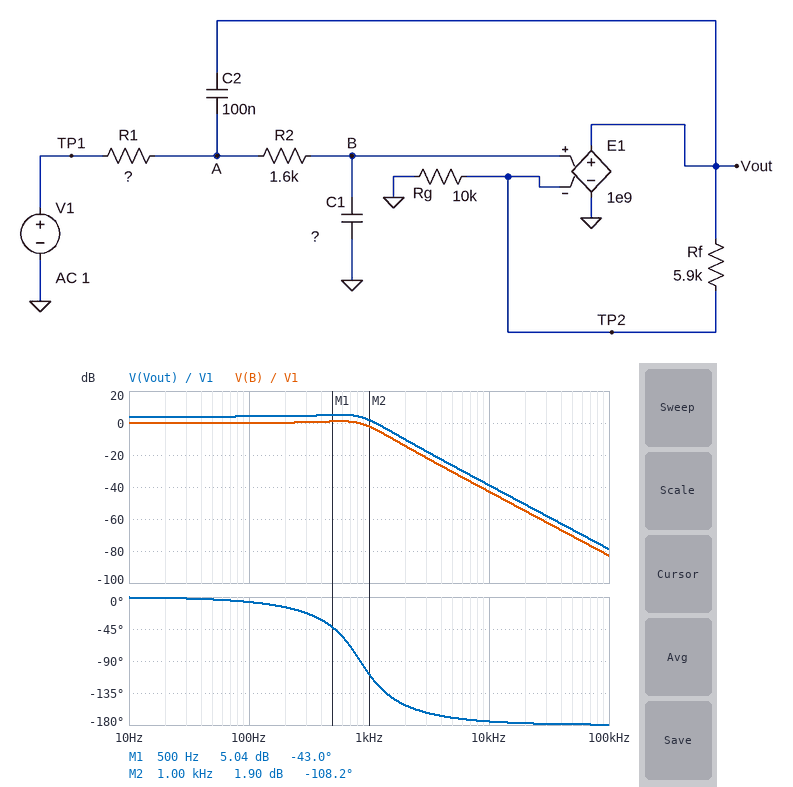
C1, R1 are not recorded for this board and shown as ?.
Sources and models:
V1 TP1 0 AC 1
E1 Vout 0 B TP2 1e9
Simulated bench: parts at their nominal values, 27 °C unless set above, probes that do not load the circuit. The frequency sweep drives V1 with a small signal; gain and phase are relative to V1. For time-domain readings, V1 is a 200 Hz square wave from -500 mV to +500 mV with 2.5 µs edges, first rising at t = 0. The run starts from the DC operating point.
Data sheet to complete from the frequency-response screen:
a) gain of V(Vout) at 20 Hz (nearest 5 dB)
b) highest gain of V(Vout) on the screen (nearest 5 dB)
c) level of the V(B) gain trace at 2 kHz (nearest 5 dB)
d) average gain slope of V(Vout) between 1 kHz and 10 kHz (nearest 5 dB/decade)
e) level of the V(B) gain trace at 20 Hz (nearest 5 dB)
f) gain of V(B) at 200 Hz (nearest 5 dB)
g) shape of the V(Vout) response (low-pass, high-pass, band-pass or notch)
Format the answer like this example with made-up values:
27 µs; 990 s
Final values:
5 dB; 5 dB; -15 dB; -40 dB/decade; 0 dB; 0 dB; low-pass
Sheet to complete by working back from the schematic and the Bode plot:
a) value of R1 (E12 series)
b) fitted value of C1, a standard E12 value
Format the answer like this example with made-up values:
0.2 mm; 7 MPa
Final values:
2.7 kΩ; 82 nF
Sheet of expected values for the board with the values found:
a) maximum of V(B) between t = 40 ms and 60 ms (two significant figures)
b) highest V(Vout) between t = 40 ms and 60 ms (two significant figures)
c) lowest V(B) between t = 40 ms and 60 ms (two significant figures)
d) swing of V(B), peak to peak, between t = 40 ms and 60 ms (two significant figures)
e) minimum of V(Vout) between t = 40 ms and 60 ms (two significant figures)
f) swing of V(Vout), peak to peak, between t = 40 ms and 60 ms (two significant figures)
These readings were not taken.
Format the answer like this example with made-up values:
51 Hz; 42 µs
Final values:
650 mV; 1.0 V; -650 mV; 1.3 V; -1.0 V; 2.1 V
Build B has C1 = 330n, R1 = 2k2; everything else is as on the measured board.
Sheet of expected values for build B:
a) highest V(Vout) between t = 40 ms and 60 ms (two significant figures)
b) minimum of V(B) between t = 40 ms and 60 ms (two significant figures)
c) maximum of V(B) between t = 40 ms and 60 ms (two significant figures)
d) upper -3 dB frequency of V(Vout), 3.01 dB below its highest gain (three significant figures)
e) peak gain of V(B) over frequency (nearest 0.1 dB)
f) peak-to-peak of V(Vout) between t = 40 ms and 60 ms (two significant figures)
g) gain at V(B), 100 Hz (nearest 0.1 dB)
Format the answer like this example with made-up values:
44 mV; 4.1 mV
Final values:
660 mV; -410 mV; 410 mV; 156 Hz; 0 dB; 1.3 V; -1.5 dB
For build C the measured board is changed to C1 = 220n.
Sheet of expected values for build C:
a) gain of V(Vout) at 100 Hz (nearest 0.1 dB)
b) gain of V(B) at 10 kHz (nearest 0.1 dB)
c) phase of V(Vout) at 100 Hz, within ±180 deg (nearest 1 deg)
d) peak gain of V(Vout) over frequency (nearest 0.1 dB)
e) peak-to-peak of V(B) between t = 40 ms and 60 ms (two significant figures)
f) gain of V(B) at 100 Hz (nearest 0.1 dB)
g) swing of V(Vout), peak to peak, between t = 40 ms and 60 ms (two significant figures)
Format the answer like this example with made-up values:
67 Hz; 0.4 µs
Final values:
3.3 dB; -51.5 dB; -27 deg; 4.0 dB; 950 mV; -0.7 dB; 1.5 V
